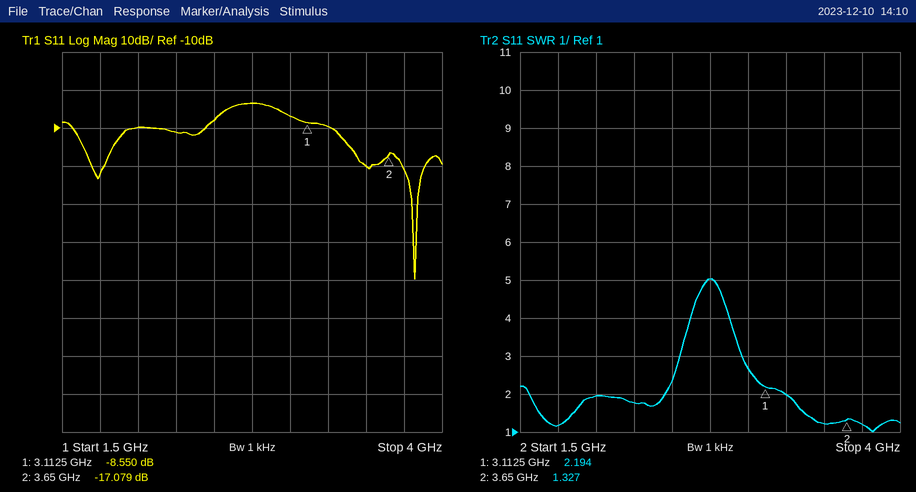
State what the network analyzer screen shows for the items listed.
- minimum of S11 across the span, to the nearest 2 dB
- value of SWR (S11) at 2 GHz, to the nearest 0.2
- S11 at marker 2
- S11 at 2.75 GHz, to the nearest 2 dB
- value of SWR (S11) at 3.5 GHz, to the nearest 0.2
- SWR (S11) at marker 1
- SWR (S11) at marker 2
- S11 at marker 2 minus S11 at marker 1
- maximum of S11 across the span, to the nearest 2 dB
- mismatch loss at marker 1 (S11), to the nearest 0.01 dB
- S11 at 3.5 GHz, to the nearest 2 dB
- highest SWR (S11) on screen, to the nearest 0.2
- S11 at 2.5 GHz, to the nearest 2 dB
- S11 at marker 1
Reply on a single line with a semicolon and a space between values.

-50 dB; 2.0; -17.079 dB; -4 dB; 1.2; 2.194; 1.327; -8.529 dB; -4 dB; 0.65 dB; -20 dB; 5.0; -8 dB; -8.550 dB
